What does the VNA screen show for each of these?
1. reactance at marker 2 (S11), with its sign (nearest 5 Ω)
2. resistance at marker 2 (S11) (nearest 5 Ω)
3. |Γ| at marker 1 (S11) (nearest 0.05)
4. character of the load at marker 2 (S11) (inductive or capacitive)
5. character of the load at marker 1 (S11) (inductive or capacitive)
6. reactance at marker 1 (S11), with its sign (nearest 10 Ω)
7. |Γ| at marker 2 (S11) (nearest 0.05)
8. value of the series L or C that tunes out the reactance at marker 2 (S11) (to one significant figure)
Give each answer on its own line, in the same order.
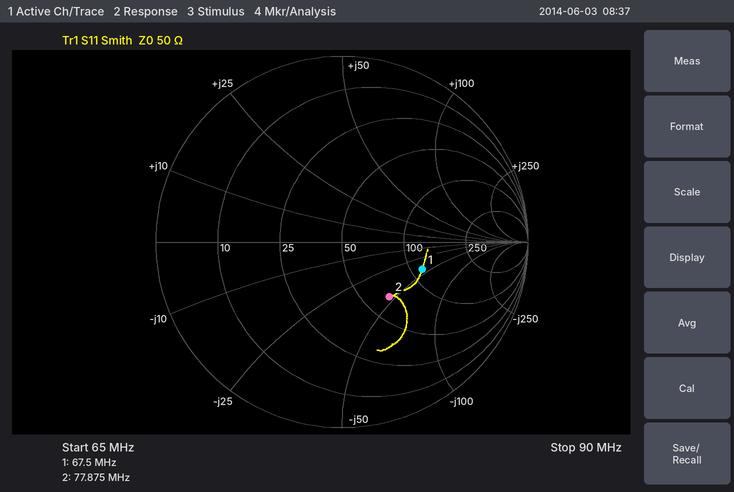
-45 Ω
65 Ω
0.45
capacitive
capacitive
-40 Ω
0.40
90 nH
